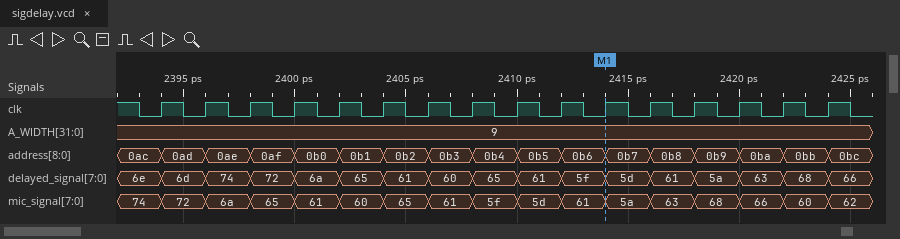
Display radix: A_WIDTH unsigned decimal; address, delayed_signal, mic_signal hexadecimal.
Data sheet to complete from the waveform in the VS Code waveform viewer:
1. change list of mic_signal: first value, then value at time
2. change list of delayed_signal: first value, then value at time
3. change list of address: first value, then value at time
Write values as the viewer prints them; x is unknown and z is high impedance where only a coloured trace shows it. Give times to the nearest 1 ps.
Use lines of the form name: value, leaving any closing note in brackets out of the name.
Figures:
change list of mic_signal: first value, then value at time: 74, 72 at 2394 ps, 6a at 2396 ps, 65 at 2398 ps, 61 at 2400 ps, 60 at 2402 ps, 65 at 2404 ps, 61 at 2406 ps, 5f at 2408 ps, 5d at 2410 ps, 61 at 2412 ps, 5a at 2414 ps, 63 at 2416 ps, 68 at 2418 ps, 66 at 2420 ps, 60 at 2422 ps, 62 at 2424 ps
change list of delayed_signal: first value, then value at time: 6e, 6d at 2394 ps, 74 at 2396 ps, 72 at 2398 ps, 6a at 2400 ps, 65 at 2402 ps, 61 at 2404 ps, 60 at 2406 ps, 65 at 2408 ps, 61 at 2410 ps, 5f at 2412 ps, 5d at 2414 ps, 61 at 2416 ps, 5a at 2418 ps, 63 at 2420 ps, 68 at 2422 ps, 66 at 2424 ps
change list of address: first value, then value at time: 0ac, 0ad at 2394 ps, 0ae at 2396 ps, 0af at 2398 ps, 0b0 at 2400 ps, 0b1 at 2402 ps, 0b2 at 2404 ps, 0b3 at 2406 ps, 0b4 at 2408 ps, 0b5 at 2410 ps, 0b6 at 2412 ps, 0b7 at 2414 ps, 0b8 at 2416 ps, 0b9 at 2418 ps, 0ba at 2420 ps, 0bb at 2422 ps, 0bc at 2424 ps
